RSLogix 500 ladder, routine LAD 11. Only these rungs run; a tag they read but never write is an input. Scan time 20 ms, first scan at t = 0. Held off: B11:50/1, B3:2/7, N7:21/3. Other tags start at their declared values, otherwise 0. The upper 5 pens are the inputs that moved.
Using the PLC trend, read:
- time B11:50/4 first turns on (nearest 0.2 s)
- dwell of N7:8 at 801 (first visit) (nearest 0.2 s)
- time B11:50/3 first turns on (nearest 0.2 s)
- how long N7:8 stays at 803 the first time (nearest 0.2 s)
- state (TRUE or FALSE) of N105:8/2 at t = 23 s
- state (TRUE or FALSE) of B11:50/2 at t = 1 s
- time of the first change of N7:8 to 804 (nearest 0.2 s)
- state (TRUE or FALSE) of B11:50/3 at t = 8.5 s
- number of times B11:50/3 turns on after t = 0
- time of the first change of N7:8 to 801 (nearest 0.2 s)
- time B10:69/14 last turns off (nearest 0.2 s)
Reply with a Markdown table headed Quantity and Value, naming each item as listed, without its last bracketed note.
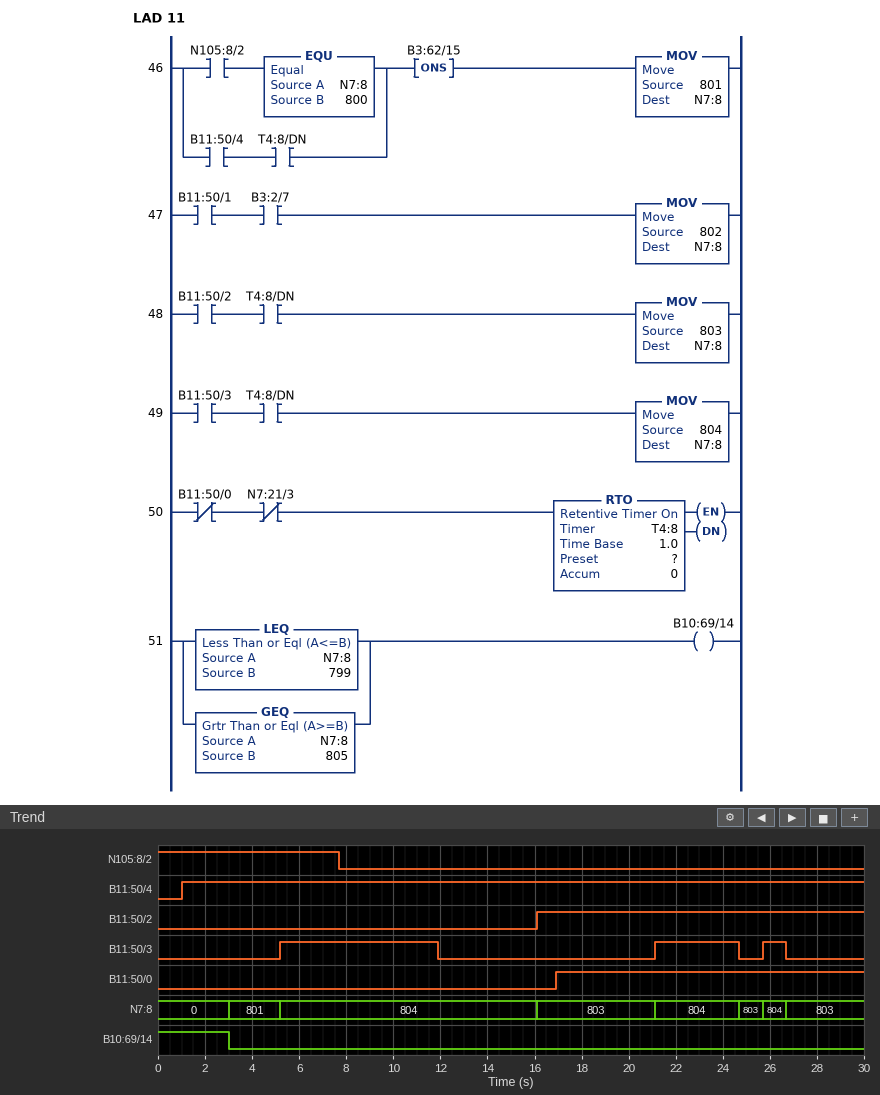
| Quantity | Value |
|---|---|
| time B11:50/4 first turns on | 1.0 s |
| dwell of N7:8 at 801 (first visit) | 2.2 s |
| time B11:50/3 first turns on | 5.2 s |
| how long N7:8 stays at 803 the first time | 5.0 s |
| state (TRUE or FALSE) of N105:8/2 at t = 23 s | FALSE |
| state (TRUE or FALSE) of B11:50/2 at t = 1 s | FALSE |
| time of the first change of N7:8 to 804 | 5.2 s |
| state (TRUE or FALSE) of B11:50/3 at t = 8.5 s | TRUE |
| number of times B11:50/3 turns on after t = 0 | 3 |
| time of the first change of N7:8 to 801 | 3.0 s |
| time B10:69/14 last turns off | 3.0 s |
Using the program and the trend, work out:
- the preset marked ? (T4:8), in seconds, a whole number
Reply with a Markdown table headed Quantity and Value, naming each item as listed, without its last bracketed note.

| Quantity | Value |
|---|---|
| the preset marked ? (T4:8), in seconds, a whole number | 3 s |
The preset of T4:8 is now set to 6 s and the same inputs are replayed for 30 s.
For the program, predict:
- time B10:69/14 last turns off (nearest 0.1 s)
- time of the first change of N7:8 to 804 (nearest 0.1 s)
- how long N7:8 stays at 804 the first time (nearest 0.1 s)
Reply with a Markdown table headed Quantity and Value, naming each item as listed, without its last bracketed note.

| Quantity | Value |
|---|---|
| time B10:69/14 last turns off | 6.0 s |
| time of the first change of N7:8 to 804 | 6.0 s |
| how long N7:8 stays at 804 the first time | 10.1 s |
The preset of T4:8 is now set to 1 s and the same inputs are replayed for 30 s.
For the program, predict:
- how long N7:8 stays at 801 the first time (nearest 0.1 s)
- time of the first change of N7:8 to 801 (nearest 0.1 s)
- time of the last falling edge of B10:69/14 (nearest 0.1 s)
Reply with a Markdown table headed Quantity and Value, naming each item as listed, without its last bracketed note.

| Quantity | Value |
|---|---|
| how long N7:8 stays at 801 the first time | 4.2 s |
| time of the first change of N7:8 to 801 | 1.0 s |
| time of the last falling edge of B10:69/14 | 1.0 s |
